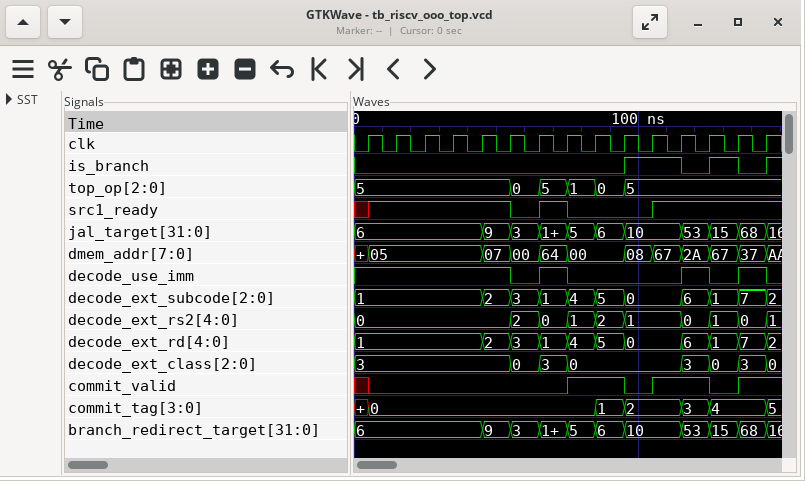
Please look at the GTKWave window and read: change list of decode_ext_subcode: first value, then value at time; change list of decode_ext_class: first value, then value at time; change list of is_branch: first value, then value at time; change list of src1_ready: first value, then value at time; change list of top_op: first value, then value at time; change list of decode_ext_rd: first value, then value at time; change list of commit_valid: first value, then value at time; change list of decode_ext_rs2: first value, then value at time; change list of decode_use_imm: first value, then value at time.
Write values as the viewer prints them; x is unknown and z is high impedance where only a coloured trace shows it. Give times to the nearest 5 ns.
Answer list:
1, 2 at 45 ns, 3 at 55 ns, 1 at 65 ns, 4 at 75 ns, 5 at 85 ns, 0 at 95 ns, 6 at 115 ns, 1 at 125 ns, 7 at 135 ns, 2 at 145 ns
3, 0 at 55 ns, 3 at 65 ns, 0 at 75 ns, 3 at 115 ns, 0 at 125 ns, 3 at 135 ns, 0 at 145 ns
0, 1 at 95 ns, 0 at 115 ns, 1 at 125 ns, 0 at 135 ns, 1 at 145 ns
x, 1 at 5 ns, 0 at 55 ns, 1 at 65 ns, 0 at 75 ns, 1 at 105 ns
5, 0 at 55 ns, 5 at 65 ns, 1 at 75 ns, 0 at 85 ns, 5 at 95 ns
1, 2 at 45 ns, 3 at 55 ns, 1 at 65 ns, 4 at 75 ns, 5 at 85 ns, 0 at 95 ns, 6 at 115 ns, 1 at 125 ns, 7 at 135 ns, 2 at 145 ns
x, 0 at 5 ns, 1 at 75 ns, 0 at 95 ns, 1 at 105 ns, 0 at 125 ns, 1 at 135 ns
0, 2 at 55 ns, 0 at 65 ns, 1 at 75 ns, 2 at 85 ns, 1 at 95 ns, 0 at 115 ns, 1 at 125 ns, 0 at 135 ns, 1 at 145 ns
1, 0 at 55 ns, 1 at 65 ns, 0 at 75 ns, 1 at 115 ns, 0 at 125 ns, 1 at 135 ns, 0 at 145 ns
